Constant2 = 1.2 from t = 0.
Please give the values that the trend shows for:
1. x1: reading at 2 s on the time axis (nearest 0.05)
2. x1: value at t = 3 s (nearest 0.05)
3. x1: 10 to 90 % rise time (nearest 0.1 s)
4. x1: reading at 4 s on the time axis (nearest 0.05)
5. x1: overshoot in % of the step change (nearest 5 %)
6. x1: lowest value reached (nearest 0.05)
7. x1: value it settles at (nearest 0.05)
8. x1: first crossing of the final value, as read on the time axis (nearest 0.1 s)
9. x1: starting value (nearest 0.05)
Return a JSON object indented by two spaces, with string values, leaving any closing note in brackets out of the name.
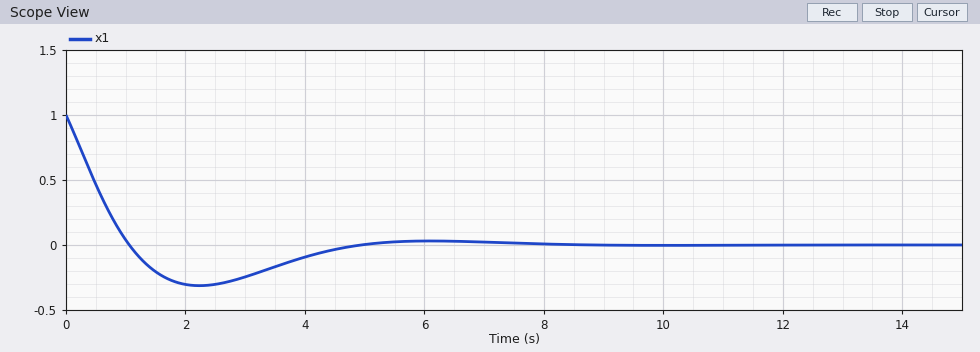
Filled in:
{
  "x1: reading at 2 s on the time axis": "-0.30",
  "x1: value at t = 3 s": "-0.25",
  "x1: 10 to 90 % rise time": "0.8 s",
  "x1: reading at 4 s on the time axis": "-0.10",
  "x1: overshoot in % of the step change": "30 %",
  "x1: lowest value reached": "-0.30",
  "x1: value it settles at": "0.00",
  "x1: first crossing of the final value, as read on the time axis": "1.1 s",
  "x1: starting value": "1.00"
}
